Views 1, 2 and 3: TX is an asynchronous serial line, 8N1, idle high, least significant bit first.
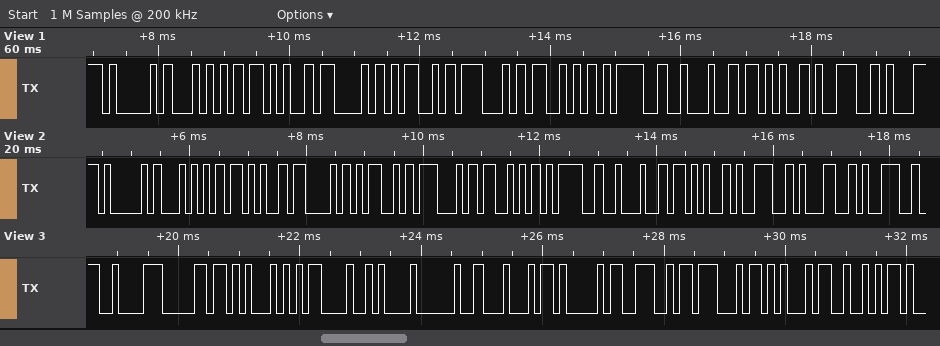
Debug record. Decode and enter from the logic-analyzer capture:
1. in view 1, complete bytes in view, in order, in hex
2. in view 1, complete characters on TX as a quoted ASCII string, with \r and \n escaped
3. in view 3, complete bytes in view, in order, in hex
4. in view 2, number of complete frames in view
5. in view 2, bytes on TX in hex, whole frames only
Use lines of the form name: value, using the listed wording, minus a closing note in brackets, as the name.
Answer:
in view 1, complete bytes in view, in order, in hex: 41 54 2B 43 4D 47 53 3D 22 2B 39
in view 1, complete characters on TX as a quoted ASCII string, with \r and \n escaped: "AT+CMGS=\"+9"
in view 3, complete bytes in view, in order, in hex: C2 B0 45 0D 0A 20 44 41 4E 47 45 52
in view 2, number of complete frames in view: 13
in view 2, bytes on TX in hex, whole frames only: 41 54 2B 43 4D 47 53 3D 22 2B 39 31 39
